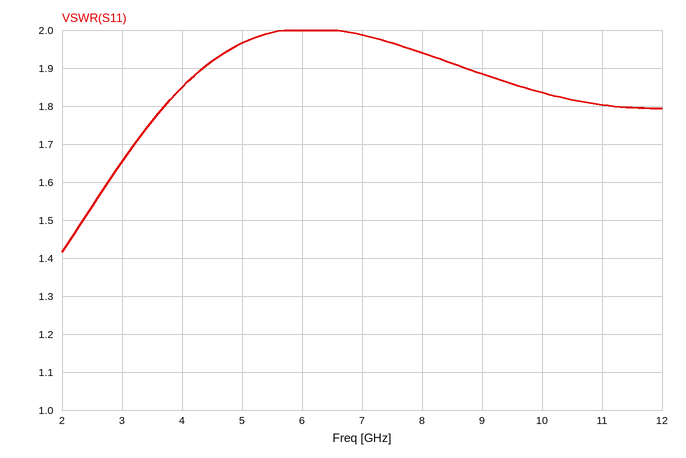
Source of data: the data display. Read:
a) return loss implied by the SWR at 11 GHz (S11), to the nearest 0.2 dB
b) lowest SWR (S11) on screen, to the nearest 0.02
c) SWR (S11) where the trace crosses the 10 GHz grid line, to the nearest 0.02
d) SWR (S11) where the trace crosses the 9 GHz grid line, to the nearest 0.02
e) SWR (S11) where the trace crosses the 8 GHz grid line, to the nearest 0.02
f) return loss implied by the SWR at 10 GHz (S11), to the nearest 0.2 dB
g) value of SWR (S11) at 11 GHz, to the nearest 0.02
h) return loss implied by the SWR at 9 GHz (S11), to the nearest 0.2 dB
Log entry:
10.8 dB
1.42
1.84
1.88
1.94
10.6 dB
1.80
10.2 dB
